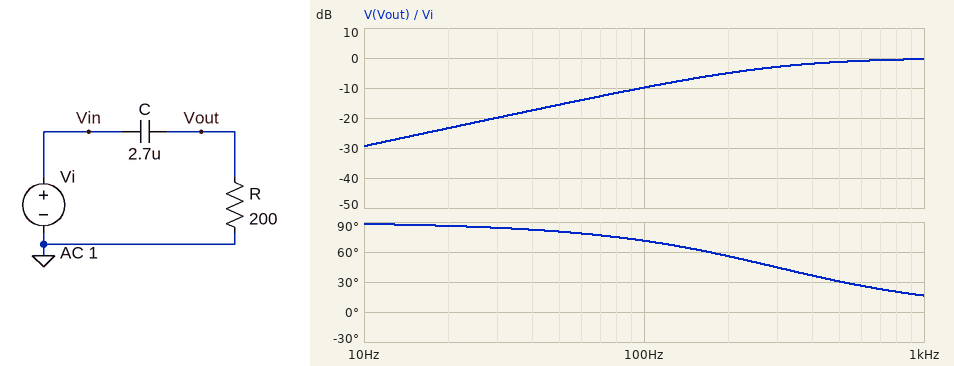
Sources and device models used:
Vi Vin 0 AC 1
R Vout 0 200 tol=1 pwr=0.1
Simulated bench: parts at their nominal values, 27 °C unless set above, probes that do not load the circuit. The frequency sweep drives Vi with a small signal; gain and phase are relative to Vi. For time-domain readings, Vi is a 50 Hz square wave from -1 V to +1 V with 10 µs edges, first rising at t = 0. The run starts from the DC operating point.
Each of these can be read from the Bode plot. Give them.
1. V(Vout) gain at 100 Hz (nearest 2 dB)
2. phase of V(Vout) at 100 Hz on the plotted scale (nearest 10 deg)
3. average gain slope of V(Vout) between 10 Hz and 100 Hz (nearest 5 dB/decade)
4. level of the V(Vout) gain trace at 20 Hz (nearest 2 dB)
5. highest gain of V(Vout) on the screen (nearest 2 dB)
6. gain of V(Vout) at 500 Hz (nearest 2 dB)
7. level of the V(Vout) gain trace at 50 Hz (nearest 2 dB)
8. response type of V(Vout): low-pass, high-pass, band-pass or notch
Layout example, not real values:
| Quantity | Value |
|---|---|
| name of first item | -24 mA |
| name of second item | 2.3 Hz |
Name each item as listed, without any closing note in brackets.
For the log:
| Quantity | Value |
|---|---|
| V(Vout) gain at 100 Hz | -10 dB |
| phase of V(Vout) at 100 Hz on the plotted scale | 70 deg |
| average gain slope of V(Vout) between 10 Hz and 100 Hz | 20 dB/decade |
| level of the V(Vout) gain trace at 20 Hz | -24 dB |
| highest gain of V(Vout) on the screen | 0 dB |
| gain of V(Vout) at 500 Hz | -2 dB |
| level of the V(Vout) gain trace at 50 Hz | -16 dB |
| response type of V(Vout): low-pass, high-pass, band-pass or notch | high-pass |
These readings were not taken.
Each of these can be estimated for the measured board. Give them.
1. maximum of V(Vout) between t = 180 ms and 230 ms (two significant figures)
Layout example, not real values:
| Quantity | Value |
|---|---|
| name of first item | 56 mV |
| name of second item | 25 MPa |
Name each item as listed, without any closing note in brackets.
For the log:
| Quantity | Value |
|---|---|
| maximum of V(Vout) between t = 180 ms and 230 ms | 2.0 V |
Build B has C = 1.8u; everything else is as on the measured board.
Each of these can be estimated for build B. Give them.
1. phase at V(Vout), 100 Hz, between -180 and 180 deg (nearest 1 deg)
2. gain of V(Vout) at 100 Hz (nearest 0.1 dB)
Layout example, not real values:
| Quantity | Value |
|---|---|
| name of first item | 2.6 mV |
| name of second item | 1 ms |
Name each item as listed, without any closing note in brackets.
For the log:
| Quantity | Value |
|---|---|
| phase at V(Vout), 100 Hz, between -180 and 180 deg | 77 deg |
| gain of V(Vout) at 100 Hz | -13.1 dB |
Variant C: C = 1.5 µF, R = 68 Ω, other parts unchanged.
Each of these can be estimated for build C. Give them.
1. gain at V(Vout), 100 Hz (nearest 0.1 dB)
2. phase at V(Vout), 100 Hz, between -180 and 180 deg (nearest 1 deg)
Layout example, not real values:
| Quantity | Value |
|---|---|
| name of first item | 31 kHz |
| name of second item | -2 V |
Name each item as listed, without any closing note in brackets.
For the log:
| Quantity | Value |
|---|---|
| gain at V(Vout), 100 Hz | -23.9 dB |
| phase at V(Vout), 100 Hz, between -180 and 180 deg | 86 deg |
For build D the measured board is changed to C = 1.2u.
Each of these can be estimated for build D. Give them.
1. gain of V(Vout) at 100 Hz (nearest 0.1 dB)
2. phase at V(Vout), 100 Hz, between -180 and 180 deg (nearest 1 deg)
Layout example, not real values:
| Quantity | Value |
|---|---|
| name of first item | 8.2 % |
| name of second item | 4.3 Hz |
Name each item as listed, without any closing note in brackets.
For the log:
| Quantity | Value |
|---|---|
| gain of V(Vout) at 100 Hz | -16.5 dB |
| phase at V(Vout), 100 Hz, between -180 and 180 deg | 81 deg |
